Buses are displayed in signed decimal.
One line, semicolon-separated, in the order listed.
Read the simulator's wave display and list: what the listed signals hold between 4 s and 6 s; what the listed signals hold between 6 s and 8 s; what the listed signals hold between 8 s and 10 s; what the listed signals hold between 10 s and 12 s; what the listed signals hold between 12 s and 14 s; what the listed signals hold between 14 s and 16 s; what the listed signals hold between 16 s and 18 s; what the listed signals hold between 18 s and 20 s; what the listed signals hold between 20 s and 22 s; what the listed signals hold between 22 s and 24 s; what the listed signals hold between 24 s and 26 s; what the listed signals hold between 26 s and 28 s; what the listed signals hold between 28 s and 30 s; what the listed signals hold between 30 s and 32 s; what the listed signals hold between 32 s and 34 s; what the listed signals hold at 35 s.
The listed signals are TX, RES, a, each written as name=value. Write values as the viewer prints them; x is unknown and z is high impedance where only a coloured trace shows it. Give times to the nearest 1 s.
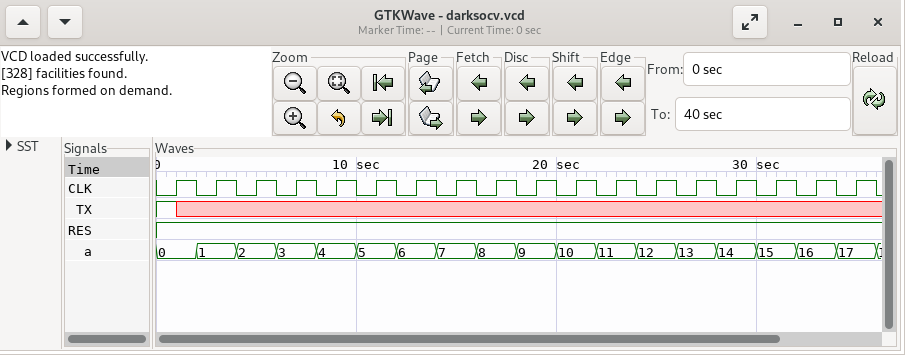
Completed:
TX=x, RES=1, a=2; TX=x, RES=1, a=3; TX=x, RES=1, a=4; TX=x, RES=1, a=5; TX=x, RES=1, a=6; TX=x, RES=1, a=7; TX=x, RES=1, a=8; TX=x, RES=1, a=9; TX=x, RES=1, a=10; TX=x, RES=1, a=11; TX=x, RES=1, a=12; TX=x, RES=1, a=13; TX=x, RES=1, a=14; TX=x, RES=1, a=15; TX=x, RES=1, a=16; TX=x, RES=1, a=17
